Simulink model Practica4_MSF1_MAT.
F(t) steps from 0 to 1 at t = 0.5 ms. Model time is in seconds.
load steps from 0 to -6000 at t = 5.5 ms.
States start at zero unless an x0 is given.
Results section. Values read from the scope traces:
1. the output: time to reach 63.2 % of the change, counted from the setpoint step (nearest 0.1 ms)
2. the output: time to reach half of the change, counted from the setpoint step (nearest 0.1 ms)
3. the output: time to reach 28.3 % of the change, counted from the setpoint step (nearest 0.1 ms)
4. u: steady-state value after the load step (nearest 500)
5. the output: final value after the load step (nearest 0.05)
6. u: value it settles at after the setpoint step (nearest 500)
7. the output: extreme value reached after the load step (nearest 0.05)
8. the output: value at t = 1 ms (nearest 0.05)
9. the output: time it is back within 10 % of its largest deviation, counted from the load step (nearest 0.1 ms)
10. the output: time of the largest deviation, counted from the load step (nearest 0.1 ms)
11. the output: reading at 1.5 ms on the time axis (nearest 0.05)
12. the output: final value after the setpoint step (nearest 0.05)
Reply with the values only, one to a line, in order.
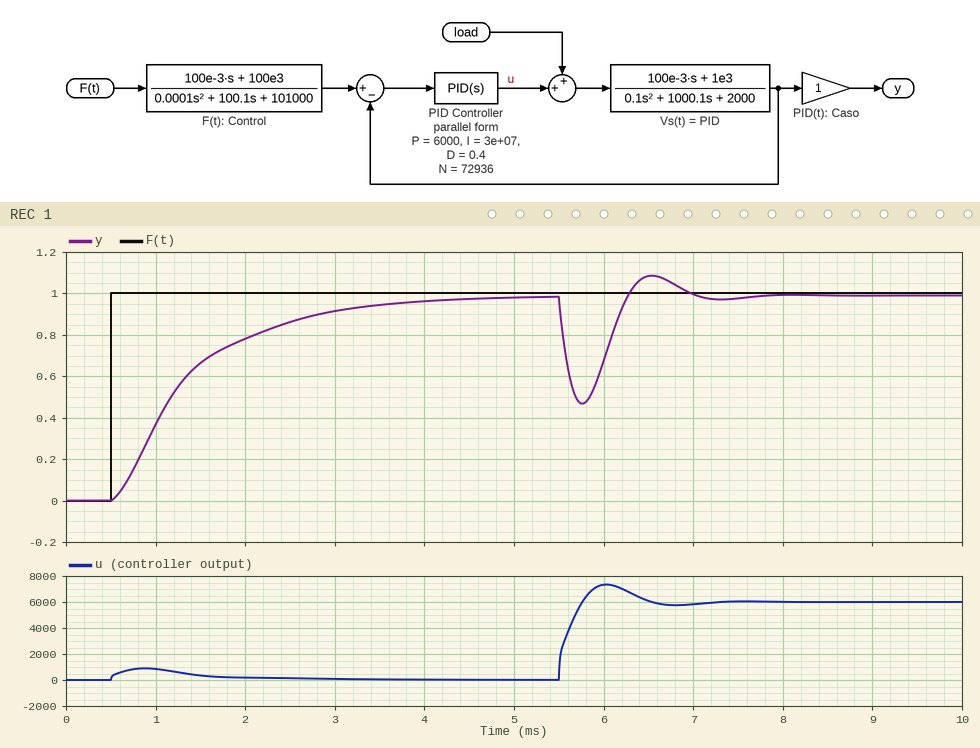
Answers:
0.9 ms
0.7 ms
0.4 ms
6000
1.00
0
0.45
0.35
1.3 ms
0.3 ms
0.65
1.00
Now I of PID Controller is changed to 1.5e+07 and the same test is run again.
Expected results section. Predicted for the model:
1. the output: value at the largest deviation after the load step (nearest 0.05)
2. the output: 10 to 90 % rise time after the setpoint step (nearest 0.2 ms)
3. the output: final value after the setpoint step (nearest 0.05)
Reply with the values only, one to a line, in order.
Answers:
0.35
2.0 ms
1.00
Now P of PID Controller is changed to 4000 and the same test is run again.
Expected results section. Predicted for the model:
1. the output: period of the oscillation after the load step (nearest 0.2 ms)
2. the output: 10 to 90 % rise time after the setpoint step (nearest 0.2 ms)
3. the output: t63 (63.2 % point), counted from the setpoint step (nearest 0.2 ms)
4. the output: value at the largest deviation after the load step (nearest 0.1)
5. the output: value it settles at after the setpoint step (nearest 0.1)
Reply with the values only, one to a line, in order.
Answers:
1.4 ms
2.0 ms
0.8 ms
0.4
1.0
